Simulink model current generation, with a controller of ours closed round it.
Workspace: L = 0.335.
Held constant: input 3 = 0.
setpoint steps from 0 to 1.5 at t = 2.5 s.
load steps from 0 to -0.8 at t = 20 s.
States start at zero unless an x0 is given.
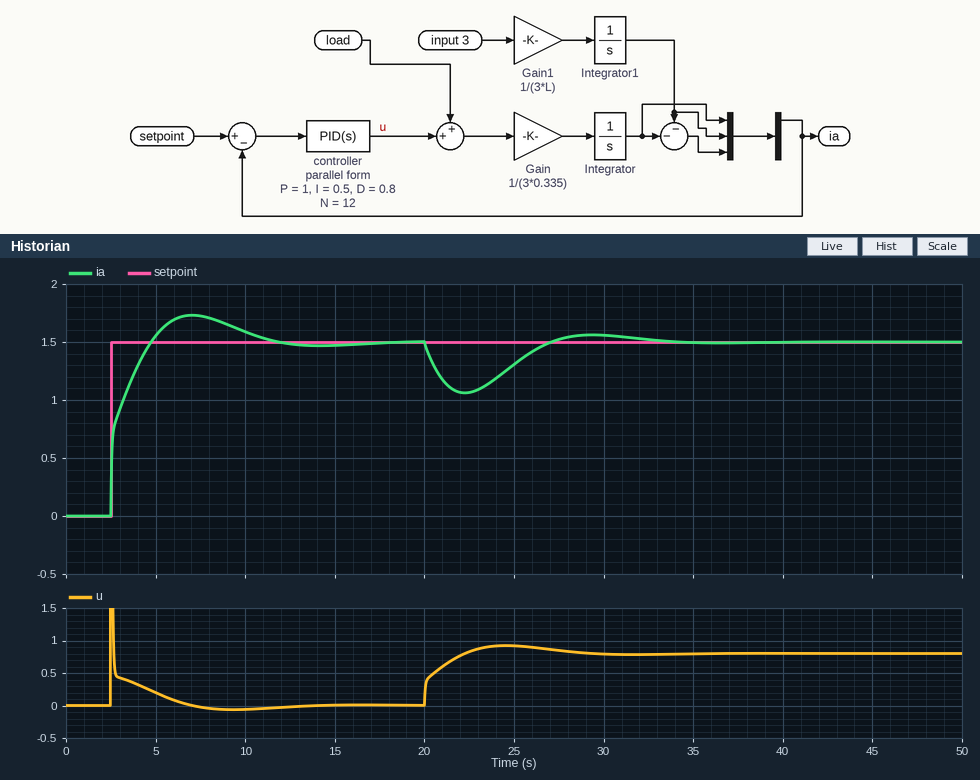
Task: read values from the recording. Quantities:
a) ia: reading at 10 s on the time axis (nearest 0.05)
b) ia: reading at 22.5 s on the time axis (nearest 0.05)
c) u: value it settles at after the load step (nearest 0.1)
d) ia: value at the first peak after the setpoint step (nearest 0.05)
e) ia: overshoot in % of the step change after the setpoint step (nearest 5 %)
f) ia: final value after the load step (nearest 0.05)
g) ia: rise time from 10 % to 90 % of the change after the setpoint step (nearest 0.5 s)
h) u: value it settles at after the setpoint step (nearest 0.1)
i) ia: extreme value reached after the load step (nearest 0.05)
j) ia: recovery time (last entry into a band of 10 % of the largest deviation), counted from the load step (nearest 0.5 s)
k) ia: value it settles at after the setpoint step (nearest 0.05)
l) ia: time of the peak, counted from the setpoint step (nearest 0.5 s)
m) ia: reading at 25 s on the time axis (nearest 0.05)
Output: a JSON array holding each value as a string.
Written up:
["1.60", "1.05", "0.8", "1.75", "15 %", "1.50", "1.5 s", "0.0", "1.05", "11.0 s", "1.50", "4.5 s", "1.30"]
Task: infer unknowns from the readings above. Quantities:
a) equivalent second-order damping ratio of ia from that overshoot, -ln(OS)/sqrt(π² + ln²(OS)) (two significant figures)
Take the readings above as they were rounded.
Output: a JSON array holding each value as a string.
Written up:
["0.52"]
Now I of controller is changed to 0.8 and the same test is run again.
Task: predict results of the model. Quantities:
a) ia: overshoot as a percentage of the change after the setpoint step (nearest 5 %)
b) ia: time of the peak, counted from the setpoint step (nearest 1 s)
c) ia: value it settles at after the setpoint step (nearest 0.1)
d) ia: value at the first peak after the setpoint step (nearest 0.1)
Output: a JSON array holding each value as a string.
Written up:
["20 %", "4 s", "1.5", "1.8"]
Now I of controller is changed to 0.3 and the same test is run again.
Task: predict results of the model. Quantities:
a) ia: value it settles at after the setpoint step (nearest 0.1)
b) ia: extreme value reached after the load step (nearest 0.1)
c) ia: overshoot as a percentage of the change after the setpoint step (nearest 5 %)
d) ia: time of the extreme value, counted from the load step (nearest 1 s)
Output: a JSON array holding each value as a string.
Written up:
["1.5", "1.0", "10 %", "3 s"]
